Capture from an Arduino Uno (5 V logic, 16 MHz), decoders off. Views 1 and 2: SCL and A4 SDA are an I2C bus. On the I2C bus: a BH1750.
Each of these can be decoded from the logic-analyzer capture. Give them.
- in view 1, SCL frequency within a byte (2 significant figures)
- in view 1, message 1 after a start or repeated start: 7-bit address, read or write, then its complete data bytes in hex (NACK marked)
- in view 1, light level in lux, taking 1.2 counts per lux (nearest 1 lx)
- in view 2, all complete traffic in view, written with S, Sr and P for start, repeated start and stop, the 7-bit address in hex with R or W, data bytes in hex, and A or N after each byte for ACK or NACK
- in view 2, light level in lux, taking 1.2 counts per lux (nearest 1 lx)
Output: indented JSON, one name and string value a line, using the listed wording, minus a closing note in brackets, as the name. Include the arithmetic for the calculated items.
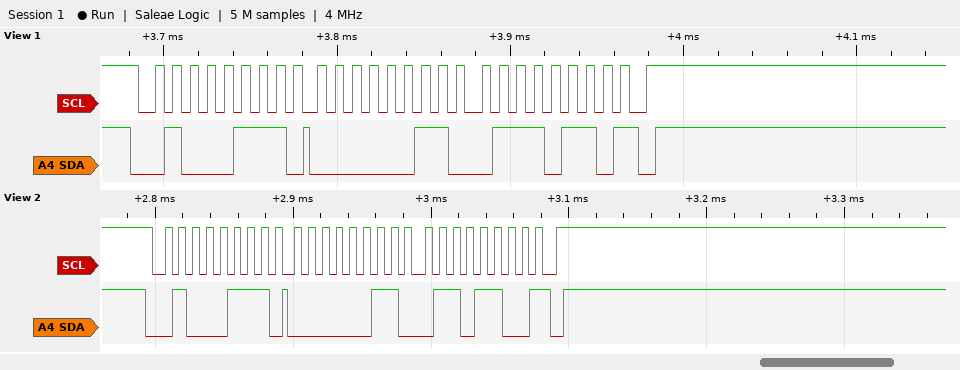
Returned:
{
  "in view 1, SCL frequency within a byte": "100 kHz",
  "in view 1, message 1 after a start or repeated start: 7-bit address, read or write, then its complete data bytes in hex": "0x23 read: 03 76 NACK",
  "in view 1, light level in lux, taking 1.2 counts per lux": "886 / 1.2 = 738 lx",
  "in view 2, all complete traffic in view, written with S, Sr and P for start, repeated start and stop, the 7-bit address in hex with R or W, data bytes in hex, and A or N after each byte for ACK or NACK": "S 23R A 03 A 6C N P",
  "in view 2, light level in lux, taking 1.2 counts per lux": "876 / 1.2 = 730 lx"
}
